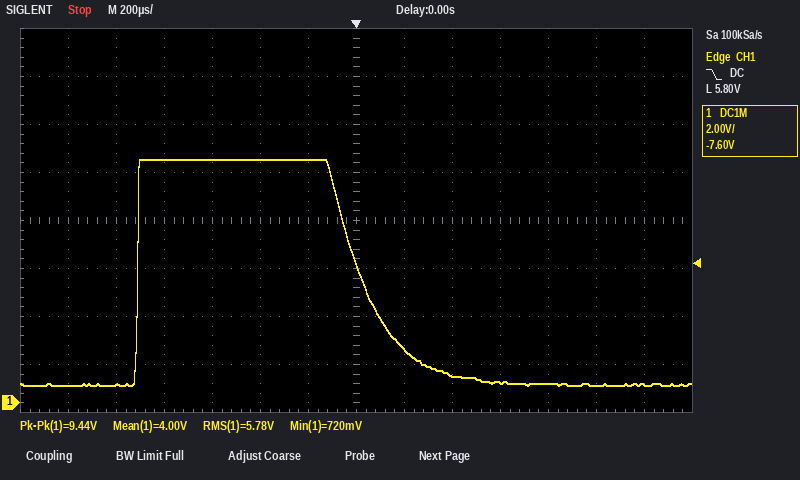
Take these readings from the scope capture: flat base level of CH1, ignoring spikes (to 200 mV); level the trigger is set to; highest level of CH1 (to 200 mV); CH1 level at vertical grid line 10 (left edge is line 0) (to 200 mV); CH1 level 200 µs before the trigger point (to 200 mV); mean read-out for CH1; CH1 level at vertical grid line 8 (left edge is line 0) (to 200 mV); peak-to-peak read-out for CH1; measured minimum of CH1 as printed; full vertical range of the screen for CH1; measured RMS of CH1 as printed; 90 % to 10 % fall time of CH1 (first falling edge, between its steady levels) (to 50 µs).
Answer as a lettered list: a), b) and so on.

a) 800 mV
b) 5.80 V
c) 10.2 V
d) 800 mV
e) 10.2 V
f) 4.00 V
g) 2.2 V
h) 9.44 V
i) 720 mV
j) 16 V
k) 5.78 V
l) 350 µs
